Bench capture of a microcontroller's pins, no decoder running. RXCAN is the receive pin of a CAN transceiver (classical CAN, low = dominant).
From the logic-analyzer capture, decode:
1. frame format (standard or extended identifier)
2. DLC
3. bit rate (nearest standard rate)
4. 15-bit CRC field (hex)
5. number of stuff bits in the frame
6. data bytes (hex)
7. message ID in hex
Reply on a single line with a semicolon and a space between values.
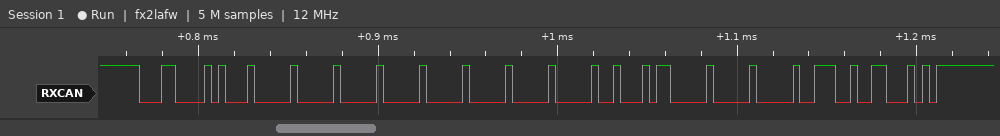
standard; 8; 250 kbit/s; 0x7262; 11; 00 00 00 00 01 16 00 00; 0x185
